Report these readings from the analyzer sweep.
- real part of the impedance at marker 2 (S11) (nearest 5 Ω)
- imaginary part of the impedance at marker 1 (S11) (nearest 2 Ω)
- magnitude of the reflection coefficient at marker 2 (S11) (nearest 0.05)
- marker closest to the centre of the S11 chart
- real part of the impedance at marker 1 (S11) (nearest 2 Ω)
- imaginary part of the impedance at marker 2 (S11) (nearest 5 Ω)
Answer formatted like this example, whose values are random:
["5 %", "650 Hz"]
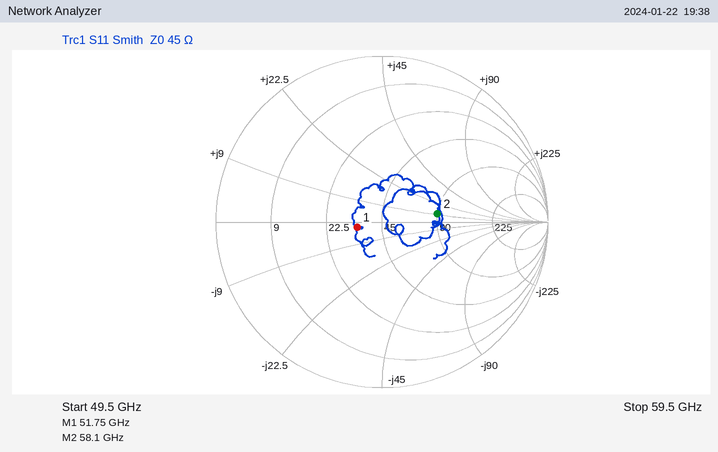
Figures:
["90 Ω", "-2 Ω", "0.35", "marker 1", "34 Ω", "+10 Ω"]
